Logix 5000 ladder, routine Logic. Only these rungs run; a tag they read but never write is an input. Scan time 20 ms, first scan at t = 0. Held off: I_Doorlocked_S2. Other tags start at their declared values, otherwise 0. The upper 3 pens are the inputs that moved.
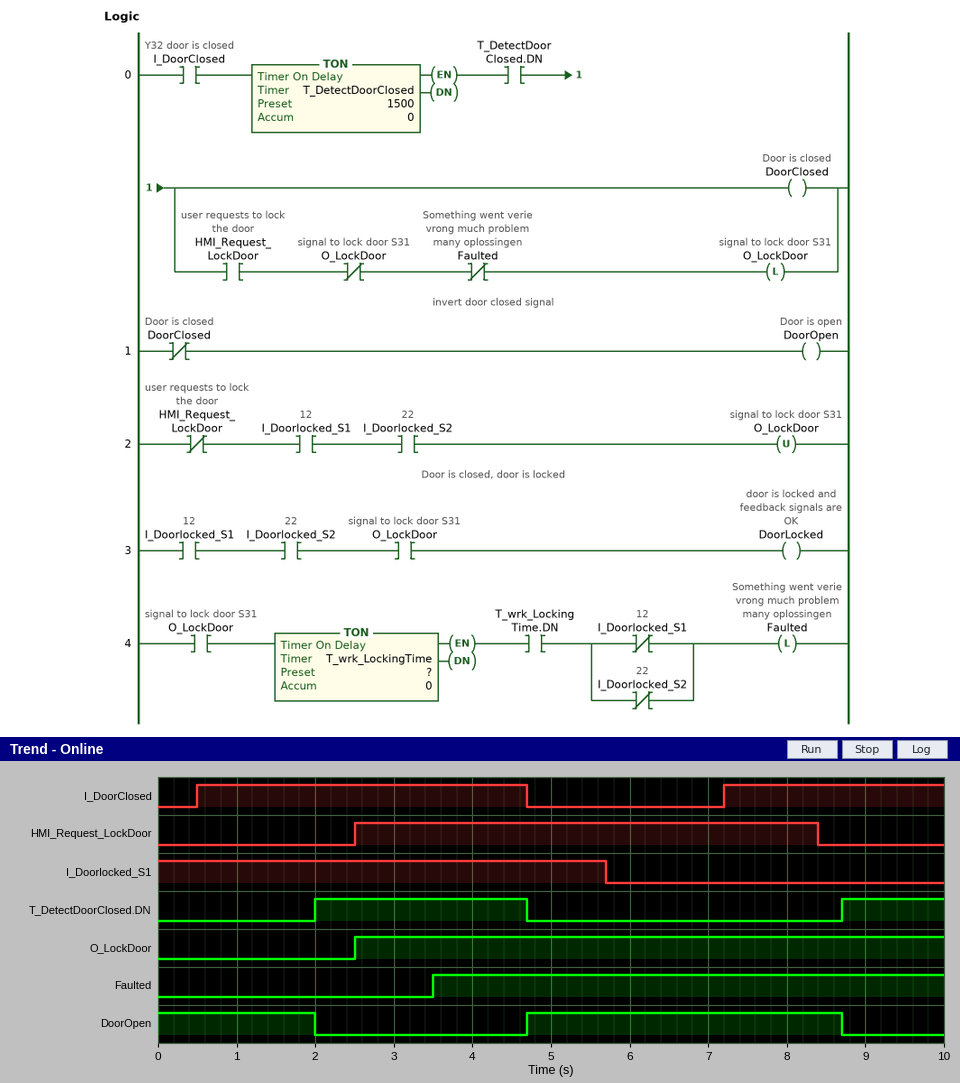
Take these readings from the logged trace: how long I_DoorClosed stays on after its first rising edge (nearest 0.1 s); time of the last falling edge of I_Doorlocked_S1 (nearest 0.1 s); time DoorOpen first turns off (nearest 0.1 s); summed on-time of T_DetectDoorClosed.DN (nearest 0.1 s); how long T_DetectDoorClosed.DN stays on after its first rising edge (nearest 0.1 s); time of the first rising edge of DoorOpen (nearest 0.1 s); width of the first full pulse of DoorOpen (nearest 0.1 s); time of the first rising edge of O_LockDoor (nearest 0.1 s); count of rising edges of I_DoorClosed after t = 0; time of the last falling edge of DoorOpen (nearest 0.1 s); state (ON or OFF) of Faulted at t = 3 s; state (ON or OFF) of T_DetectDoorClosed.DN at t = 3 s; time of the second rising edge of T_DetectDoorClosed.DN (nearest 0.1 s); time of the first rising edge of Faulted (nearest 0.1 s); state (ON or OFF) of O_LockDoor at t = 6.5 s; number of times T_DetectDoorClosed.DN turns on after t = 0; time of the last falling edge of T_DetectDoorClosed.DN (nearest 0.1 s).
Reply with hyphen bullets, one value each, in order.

- 4.2 s
- 5.7 s
- 2.0 s
- 4.0 s
- 2.7 s
- 4.7 s
- 4.0 s
- 2.5 s
- 2
- 8.7 s
- OFF
- ON
- 8.7 s
- 3.5 s
- ON
- 2
- 4.7 s
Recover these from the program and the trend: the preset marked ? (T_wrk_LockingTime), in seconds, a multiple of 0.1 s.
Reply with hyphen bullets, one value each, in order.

- 1.0 s
